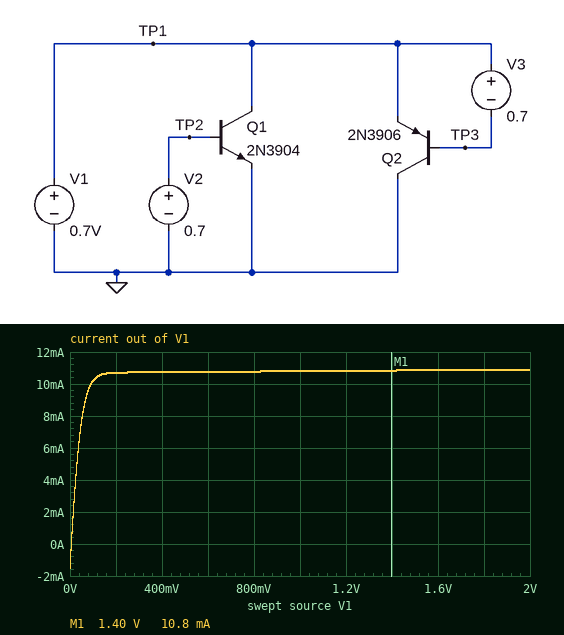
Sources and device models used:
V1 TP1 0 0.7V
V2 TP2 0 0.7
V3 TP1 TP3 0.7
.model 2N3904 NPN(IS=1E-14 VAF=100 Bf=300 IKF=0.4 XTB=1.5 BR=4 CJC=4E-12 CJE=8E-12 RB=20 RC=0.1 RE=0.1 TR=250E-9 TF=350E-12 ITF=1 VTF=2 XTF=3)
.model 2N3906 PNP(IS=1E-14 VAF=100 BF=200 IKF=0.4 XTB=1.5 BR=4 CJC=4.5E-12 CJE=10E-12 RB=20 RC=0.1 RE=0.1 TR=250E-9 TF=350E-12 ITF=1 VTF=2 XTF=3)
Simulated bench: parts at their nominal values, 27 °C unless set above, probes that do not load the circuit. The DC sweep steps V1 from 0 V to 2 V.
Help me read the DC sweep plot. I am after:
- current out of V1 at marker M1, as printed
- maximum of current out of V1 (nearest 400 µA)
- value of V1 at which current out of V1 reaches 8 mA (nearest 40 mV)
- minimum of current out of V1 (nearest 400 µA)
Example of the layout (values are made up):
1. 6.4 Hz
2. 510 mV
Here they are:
1. 10.8 mA
2. 10.8 mA
3. 40 mV
4. -1.6 mA
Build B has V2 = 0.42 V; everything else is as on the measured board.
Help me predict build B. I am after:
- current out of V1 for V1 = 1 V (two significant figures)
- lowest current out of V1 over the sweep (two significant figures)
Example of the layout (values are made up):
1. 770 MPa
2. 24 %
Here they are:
1. 5.4 mA
2. -760 µA
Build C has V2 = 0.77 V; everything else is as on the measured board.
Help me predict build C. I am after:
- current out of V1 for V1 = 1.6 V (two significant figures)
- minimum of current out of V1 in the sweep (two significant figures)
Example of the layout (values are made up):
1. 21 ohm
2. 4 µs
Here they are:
1. 58 mA
2. -3.3 mA
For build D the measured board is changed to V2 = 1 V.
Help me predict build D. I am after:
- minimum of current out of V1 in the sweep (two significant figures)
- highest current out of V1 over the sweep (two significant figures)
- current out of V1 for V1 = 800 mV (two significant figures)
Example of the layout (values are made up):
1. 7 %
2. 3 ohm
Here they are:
1. -11 mA
2. 600 mA
3. 590 mA
